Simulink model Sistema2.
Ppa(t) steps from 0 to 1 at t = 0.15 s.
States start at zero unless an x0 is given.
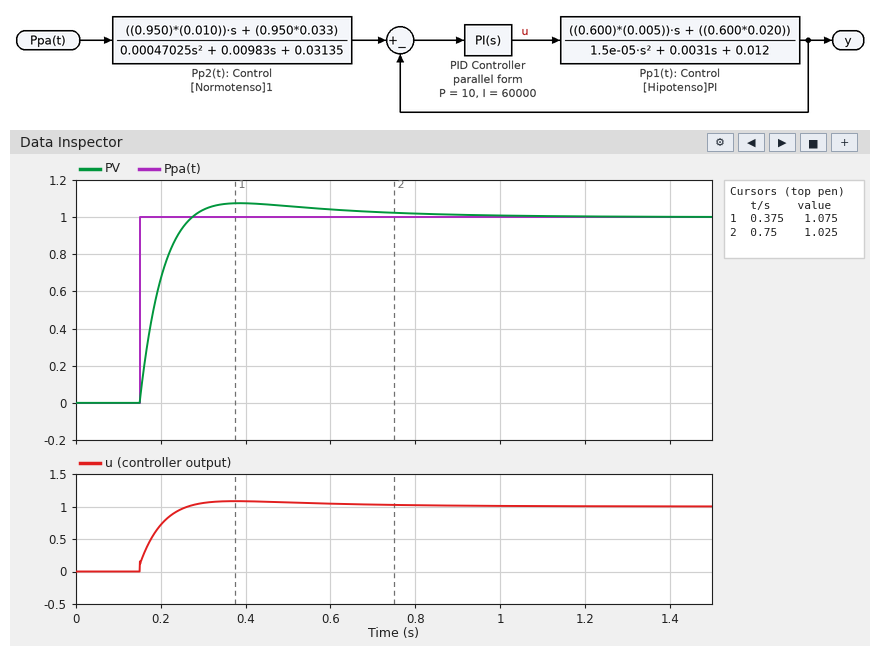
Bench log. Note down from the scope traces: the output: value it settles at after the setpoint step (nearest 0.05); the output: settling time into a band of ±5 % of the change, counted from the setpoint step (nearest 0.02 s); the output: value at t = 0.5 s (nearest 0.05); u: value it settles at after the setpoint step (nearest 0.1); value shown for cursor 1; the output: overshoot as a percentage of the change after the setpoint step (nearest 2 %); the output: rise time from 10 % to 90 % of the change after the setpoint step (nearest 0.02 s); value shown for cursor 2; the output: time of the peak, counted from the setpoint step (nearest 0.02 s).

1.00
0.40 s
1.05
1.0
1.075
8 %
0.08 s
1.025
0.24 s
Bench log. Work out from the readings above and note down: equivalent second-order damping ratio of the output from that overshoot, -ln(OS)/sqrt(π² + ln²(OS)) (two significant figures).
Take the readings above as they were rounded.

0.63
